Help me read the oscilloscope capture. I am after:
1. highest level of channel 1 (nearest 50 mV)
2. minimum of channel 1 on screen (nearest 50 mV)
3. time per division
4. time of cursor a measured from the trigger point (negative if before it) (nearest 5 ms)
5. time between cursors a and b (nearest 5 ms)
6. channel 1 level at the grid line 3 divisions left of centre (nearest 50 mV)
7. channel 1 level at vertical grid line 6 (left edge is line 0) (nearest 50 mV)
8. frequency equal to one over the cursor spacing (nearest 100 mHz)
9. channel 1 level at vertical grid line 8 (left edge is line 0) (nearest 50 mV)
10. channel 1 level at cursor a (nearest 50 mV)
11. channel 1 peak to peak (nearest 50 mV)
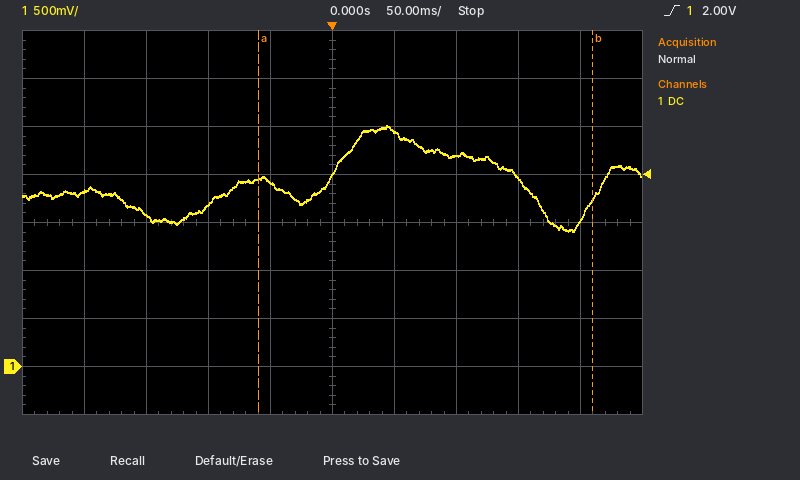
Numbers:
2.50 V
1.40 V
50 ms
-60 ms
270 ms
1.60 V
2.45 V
3.7 Hz
1.95 V
1.95 V
1.10 V
